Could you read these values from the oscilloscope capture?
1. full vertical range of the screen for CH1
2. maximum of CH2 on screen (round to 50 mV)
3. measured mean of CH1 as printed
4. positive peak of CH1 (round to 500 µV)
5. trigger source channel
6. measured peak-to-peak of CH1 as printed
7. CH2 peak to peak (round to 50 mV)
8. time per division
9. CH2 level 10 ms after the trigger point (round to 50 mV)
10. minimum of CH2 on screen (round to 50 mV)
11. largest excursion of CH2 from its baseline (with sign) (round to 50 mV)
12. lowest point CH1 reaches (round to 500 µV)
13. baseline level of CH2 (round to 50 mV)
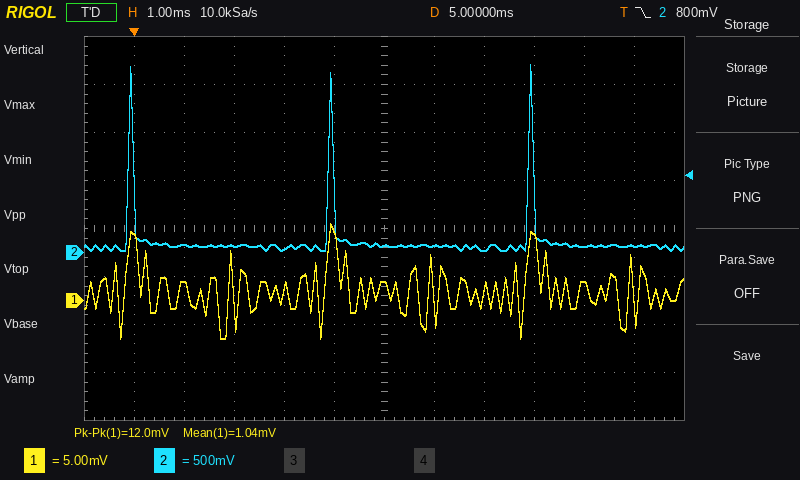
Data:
40 mV
1.95 V
1.04 mV
8.0 mV
CH2
12.0 mV
1.95 V
1 ms
50 mV
0 mV
+1.90 V
-4.0 mV
50 mV
